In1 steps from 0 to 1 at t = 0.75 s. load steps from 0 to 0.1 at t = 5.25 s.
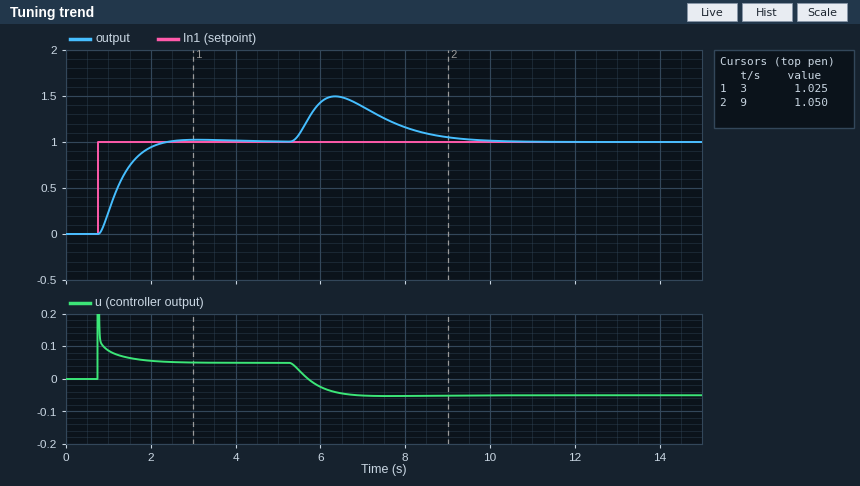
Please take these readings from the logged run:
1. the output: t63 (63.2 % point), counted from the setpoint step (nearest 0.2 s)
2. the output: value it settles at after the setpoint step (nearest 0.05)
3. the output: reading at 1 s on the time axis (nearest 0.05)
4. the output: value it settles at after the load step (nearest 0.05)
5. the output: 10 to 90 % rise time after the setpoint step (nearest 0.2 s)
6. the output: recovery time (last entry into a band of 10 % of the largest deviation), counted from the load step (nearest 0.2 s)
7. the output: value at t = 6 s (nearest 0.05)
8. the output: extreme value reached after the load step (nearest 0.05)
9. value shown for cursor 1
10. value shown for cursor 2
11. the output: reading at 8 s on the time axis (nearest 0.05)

0.6 s
1.00
0.25
1.00
1.0 s
3.8 s
1.45
1.50
1.025
1.050
1.15
